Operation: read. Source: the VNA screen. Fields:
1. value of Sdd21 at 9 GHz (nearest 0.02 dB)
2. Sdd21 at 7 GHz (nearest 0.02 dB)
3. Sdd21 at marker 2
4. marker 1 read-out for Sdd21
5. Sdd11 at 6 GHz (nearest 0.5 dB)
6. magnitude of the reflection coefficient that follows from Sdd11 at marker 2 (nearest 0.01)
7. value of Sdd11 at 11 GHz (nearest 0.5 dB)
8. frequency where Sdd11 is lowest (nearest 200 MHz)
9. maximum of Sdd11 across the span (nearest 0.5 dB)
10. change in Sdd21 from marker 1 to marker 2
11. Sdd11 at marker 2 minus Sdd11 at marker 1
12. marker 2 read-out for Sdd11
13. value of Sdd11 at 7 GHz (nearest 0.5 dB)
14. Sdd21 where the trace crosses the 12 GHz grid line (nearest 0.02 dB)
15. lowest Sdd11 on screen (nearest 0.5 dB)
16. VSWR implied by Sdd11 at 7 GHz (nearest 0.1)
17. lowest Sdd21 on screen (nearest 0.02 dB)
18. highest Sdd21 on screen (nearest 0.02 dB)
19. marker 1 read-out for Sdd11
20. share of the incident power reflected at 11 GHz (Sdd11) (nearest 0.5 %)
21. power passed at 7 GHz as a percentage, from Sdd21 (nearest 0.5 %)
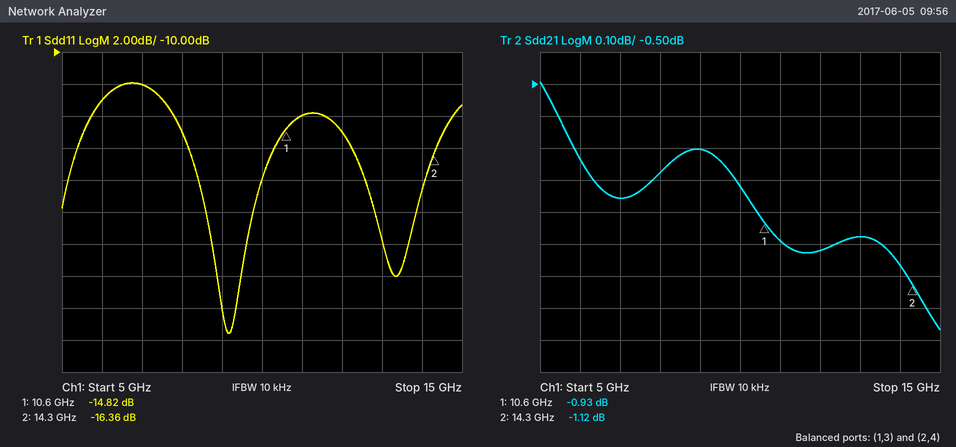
-0.70 dB
-0.86 dB
-1.12 dB
-0.93 dB
-13.0 dB
0.15
-14.0 dB
9.2 GHz
-12.0 dB
-0.19 dB
-1.54 dB
-16.36 dB
-12.0 dB
-1.02 dB
-27.5 dB
1.7
-1.26 dB
-0.50 dB
-14.82 dB
4.0 %
82.0 %
